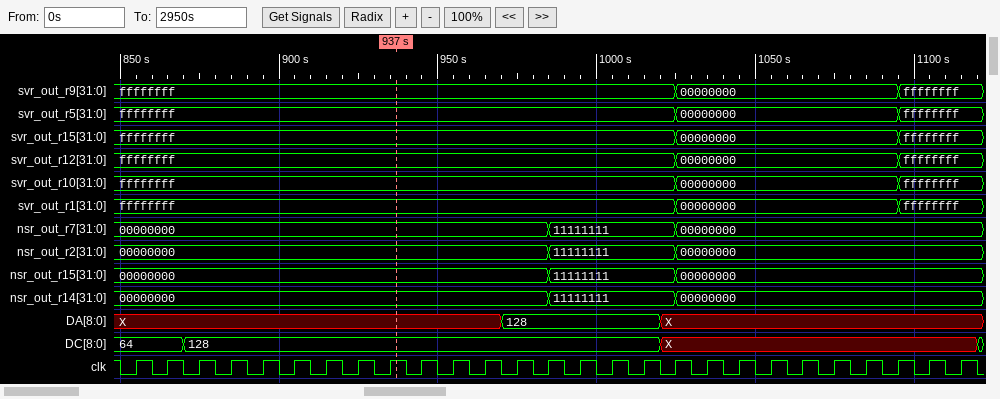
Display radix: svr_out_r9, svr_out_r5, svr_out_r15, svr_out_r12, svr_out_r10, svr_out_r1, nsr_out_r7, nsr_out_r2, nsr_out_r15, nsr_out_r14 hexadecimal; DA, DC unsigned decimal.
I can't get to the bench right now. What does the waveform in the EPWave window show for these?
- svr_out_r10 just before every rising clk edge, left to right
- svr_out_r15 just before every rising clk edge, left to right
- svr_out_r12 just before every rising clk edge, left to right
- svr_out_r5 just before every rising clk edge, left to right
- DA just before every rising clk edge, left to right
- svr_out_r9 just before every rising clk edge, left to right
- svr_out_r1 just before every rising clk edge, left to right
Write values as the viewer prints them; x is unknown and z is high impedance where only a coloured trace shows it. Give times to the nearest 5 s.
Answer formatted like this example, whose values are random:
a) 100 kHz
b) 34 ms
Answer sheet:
a) ffffffff, ffffffff, ffffffff, ffffffff, ffffffff, ffffffff, ffffffff, ffffffff, ffffffff, ffffffff, ffffffff, ffffffff, ffffffff, ffffffff, ffffffff, ffffffff, ffffffff, ffffffff, 00000000, 00000000, 00000000, 00000000, 00000000, 00000000, 00000000, ffffffff, ffffffff
b) ffffffff, ffffffff, ffffffff, ffffffff, ffffffff, ffffffff, ffffffff, ffffffff, ffffffff, ffffffff, ffffffff, ffffffff, ffffffff, ffffffff, ffffffff, ffffffff, ffffffff, ffffffff, 00000000, 00000000, 00000000, 00000000, 00000000, 00000000, 00000000, ffffffff, ffffffff
c) ffffffff, ffffffff, ffffffff, ffffffff, ffffffff, ffffffff, ffffffff, ffffffff, ffffffff, ffffffff, ffffffff, ffffffff, ffffffff, ffffffff, ffffffff, ffffffff, ffffffff, ffffffff, 00000000, 00000000, 00000000, 00000000, 00000000, 00000000, 00000000, ffffffff, ffffffff
d) ffffffff, ffffffff, ffffffff, ffffffff, ffffffff, ffffffff, ffffffff, ffffffff, ffffffff, ffffffff, ffffffff, ffffffff, ffffffff, ffffffff, ffffffff, ffffffff, ffffffff, ffffffff, 00000000, 00000000, 00000000, 00000000, 00000000, 00000000, 00000000, ffffffff, ffffffff
e) X, X, X, X, X, X, X, X, X, X, X, X, 128, 128, 128, 128, 128, X, X, X, X, X, X, X, X, X, X
f) ffffffff, ffffffff, ffffffff, ffffffff, ffffffff, ffffffff, ffffffff, ffffffff, ffffffff, ffffffff, ffffffff, ffffffff, ffffffff, ffffffff, ffffffff, ffffffff, ffffffff, ffffffff, 00000000, 00000000, 00000000, 00000000, 00000000, 00000000, 00000000, ffffffff, ffffffff
g) ffffffff, ffffffff, ffffffff, ffffffff, ffffffff, ffffffff, ffffffff, ffffffff, ffffffff, ffffffff, ffffffff, ffffffff, ffffffff, ffffffff, ffffffff, ffffffff, ffffffff, ffffffff, 00000000, 00000000, 00000000, 00000000, 00000000, 00000000, 00000000, ffffffff, ffffffff
